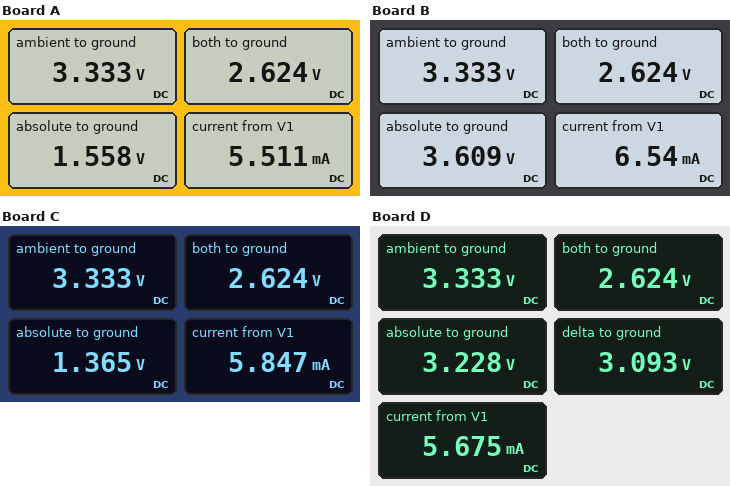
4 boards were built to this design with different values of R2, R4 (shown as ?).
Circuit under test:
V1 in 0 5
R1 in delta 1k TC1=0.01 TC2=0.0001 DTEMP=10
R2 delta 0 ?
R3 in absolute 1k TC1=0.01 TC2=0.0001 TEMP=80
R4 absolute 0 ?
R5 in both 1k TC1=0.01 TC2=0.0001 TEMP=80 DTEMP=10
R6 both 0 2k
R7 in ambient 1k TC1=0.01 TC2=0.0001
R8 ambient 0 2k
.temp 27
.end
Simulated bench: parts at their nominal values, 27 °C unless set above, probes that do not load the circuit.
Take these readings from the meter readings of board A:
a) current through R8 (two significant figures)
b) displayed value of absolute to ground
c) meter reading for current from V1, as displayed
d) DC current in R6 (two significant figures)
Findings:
1.7 mA
1.558 V
5.511 mA
1.3 mA
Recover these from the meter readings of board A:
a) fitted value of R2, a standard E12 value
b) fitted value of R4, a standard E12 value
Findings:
6.8 kΩ
820 Ω
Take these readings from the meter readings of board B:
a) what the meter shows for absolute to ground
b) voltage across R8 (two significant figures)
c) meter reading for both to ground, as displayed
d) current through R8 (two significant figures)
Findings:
3.609 V
3.3 V
2.624 V
1.7 mA
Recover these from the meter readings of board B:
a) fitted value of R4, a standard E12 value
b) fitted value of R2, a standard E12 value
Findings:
4.7 kΩ
680 Ω
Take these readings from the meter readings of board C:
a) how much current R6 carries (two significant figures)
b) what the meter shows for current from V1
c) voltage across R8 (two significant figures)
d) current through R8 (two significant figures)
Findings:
1.3 mA
5.847 mA
3.3 V
1.7 mA
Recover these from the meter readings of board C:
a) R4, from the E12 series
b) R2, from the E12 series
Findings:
680 Ω
4.7 kΩ
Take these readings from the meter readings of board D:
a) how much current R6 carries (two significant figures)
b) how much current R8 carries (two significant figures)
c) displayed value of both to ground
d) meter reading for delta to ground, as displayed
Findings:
1.3 mA
1.7 mA
2.624 V
3.093 V
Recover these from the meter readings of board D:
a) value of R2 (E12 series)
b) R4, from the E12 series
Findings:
1.8 kΩ
3.3 kΩ
